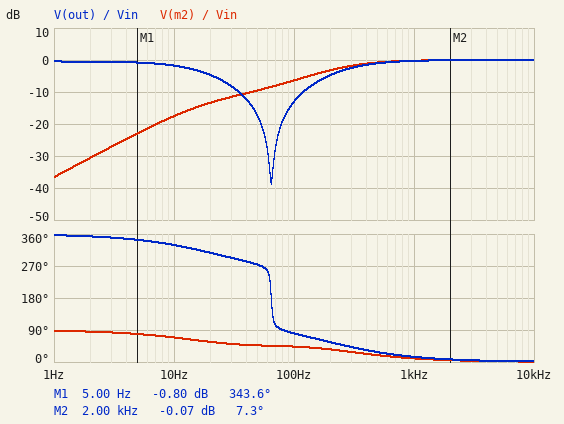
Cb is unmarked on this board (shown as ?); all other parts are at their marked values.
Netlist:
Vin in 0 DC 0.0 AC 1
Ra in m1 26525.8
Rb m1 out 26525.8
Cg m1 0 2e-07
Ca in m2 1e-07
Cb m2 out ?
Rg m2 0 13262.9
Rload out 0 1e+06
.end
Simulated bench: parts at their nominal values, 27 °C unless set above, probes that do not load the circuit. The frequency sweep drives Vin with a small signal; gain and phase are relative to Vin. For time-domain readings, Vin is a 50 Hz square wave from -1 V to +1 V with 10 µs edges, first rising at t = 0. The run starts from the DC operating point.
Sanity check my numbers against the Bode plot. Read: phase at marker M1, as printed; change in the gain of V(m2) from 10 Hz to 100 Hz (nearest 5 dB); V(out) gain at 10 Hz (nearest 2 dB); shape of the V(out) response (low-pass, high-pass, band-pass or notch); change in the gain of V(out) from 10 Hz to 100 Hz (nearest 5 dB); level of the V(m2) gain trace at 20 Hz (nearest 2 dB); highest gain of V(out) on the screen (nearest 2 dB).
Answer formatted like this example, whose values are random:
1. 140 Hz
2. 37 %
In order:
1. 343.6 deg
2. 10 dB
3. -2 dB
4. notch
5. -10 dB
6. -14 dB
7. 0 dB
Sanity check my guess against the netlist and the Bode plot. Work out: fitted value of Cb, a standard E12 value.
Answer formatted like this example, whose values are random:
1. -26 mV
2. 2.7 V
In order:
1. 82 nF
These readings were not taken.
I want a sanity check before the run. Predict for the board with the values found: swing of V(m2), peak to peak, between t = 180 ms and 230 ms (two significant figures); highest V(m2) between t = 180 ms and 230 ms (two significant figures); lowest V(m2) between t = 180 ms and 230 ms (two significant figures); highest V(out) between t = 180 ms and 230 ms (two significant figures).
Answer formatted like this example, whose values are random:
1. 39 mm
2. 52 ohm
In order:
1. 3.8 V
2. 1.9 V
3. -1.9 V
4. 1.6 V
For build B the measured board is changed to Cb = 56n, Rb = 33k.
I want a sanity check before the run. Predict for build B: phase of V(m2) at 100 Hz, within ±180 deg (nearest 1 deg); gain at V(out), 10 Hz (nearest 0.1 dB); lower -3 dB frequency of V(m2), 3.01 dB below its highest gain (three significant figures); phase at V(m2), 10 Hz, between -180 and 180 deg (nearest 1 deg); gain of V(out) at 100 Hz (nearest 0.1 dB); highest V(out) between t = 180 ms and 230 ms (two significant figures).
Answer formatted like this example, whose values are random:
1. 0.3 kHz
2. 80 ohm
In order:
1. 44 deg
2. -1.5 dB
3. 192 Hz
4. 74 deg
5. -13.5 dB
6. 1.5 V
